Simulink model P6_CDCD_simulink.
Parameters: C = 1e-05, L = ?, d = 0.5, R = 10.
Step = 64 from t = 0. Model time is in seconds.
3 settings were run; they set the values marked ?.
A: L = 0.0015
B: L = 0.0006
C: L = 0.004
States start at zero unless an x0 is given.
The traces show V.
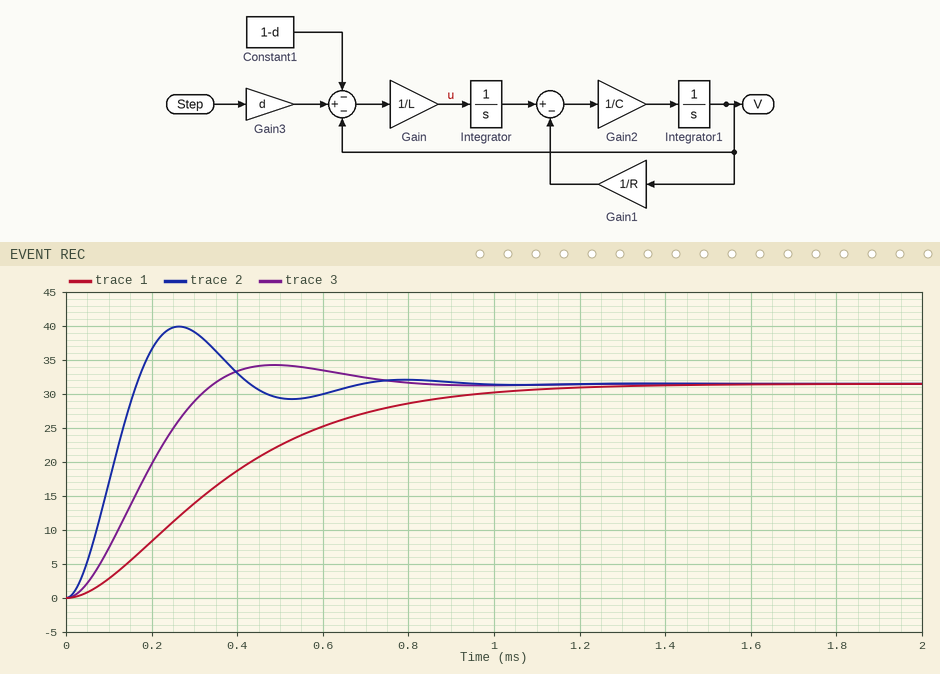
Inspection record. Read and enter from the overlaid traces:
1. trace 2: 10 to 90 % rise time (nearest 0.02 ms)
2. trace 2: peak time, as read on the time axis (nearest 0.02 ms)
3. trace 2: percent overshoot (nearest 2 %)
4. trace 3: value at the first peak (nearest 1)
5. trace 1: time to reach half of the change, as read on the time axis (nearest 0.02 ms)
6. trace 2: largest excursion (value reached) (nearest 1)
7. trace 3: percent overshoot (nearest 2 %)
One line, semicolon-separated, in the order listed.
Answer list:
0.12 ms; 0.26 ms; 26 %; 34; 0.34 ms; 40; 8 %
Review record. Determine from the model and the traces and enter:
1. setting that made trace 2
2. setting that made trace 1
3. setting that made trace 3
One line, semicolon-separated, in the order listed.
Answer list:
B; C; A
